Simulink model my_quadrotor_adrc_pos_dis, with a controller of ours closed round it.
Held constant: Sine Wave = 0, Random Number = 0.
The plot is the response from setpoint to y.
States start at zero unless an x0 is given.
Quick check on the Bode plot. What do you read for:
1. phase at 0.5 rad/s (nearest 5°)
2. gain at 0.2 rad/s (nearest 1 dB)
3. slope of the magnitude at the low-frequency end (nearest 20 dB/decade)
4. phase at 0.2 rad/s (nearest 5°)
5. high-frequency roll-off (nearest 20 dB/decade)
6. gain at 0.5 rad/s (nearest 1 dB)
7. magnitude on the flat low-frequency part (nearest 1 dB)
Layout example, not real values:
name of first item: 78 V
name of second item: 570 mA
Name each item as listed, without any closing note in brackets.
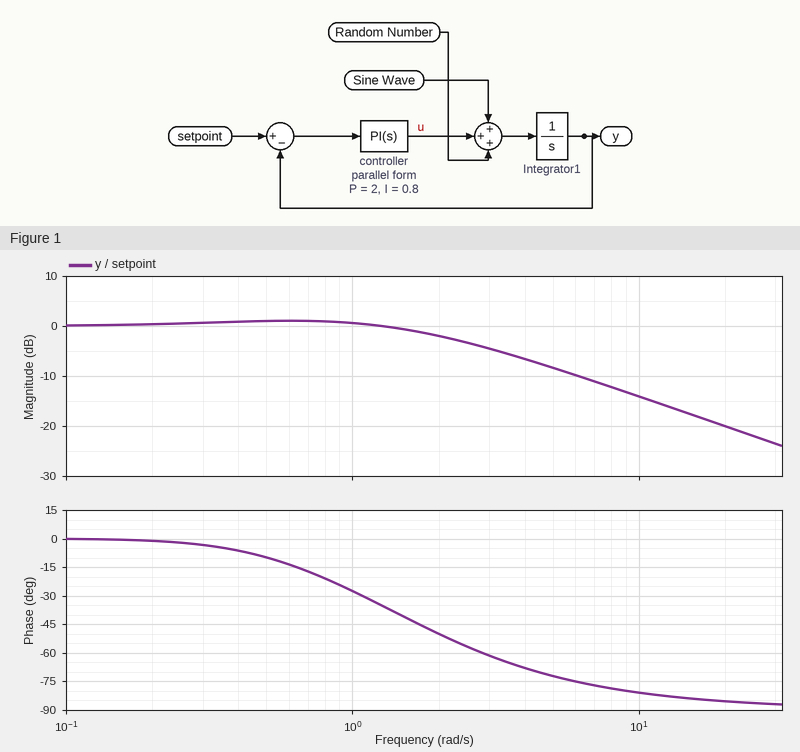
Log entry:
phase at 0.5 rad/s: -10°
gain at 0.2 rad/s: 0 dB
slope of the magnitude at the low-frequency end: 0 dB/decade
phase at 0.2 rad/s: 0°
high-frequency roll-off: -20 dB/decade
gain at 0.5 rad/s: 1 dB
magnitude on the flat low-frequency part: 0 dB
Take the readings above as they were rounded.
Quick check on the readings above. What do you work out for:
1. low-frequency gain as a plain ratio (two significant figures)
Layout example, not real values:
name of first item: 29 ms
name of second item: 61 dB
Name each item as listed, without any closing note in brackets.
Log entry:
low-frequency gain as a plain ratio: 1.0
